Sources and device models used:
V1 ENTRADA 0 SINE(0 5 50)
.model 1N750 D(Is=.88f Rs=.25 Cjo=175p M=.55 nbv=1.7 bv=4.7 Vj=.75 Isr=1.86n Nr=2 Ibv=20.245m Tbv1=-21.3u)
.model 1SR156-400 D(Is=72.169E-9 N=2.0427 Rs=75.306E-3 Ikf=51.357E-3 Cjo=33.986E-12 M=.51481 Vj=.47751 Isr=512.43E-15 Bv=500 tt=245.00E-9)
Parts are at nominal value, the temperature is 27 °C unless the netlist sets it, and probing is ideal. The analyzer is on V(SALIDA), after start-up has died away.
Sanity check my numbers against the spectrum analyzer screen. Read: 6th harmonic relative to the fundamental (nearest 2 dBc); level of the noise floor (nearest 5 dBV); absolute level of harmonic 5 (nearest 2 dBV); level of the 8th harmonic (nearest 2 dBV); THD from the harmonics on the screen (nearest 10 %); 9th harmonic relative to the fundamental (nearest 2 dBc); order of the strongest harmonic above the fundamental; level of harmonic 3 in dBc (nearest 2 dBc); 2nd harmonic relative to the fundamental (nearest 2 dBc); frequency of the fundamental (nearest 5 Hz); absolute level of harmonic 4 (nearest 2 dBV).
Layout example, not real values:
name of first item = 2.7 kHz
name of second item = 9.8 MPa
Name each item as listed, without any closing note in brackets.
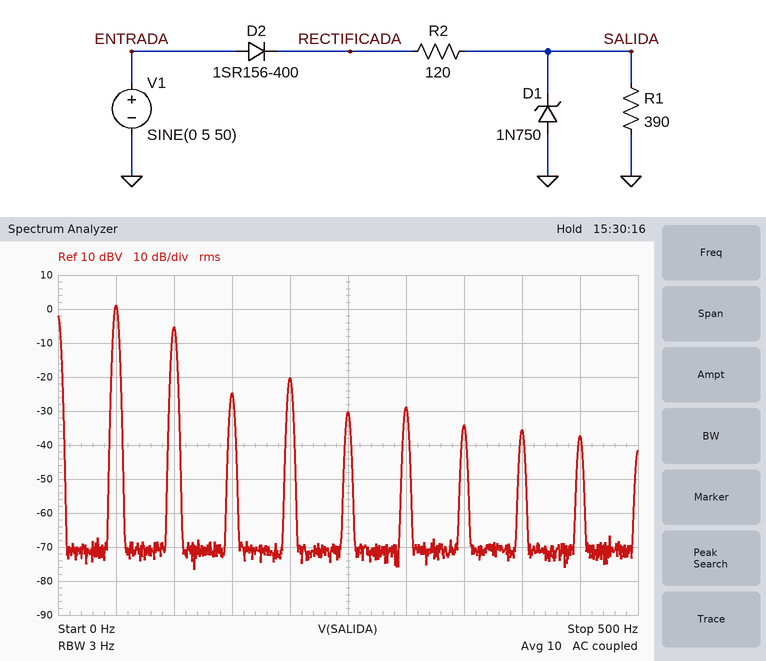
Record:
6th harmonic relative to the fundamental = -30 dBc
level of the noise floor = -70 dBV
absolute level of harmonic 5 = -30 dBV
level of the 8th harmonic = -36 dBV
THD from the harmonics on the screen = 50 %
9th harmonic relative to the fundamental = -38 dBc
order of the strongest harmonic above the fundamental = 2
level of harmonic 3 in dBc = -26 dBc
2nd harmonic relative to the fundamental = -6 dBc
frequency of the fundamental = 50 Hz
absolute level of harmonic 4 = -20 dBV
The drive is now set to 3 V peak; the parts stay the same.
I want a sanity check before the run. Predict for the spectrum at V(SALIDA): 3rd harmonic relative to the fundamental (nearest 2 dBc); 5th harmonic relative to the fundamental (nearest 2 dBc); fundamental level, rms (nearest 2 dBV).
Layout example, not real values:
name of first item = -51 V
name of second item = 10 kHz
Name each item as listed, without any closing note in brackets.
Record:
3rd harmonic relative to the fundamental = -22 dBc
5th harmonic relative to the fundamental = -28 dBc
fundamental level, rms = -4 dBV
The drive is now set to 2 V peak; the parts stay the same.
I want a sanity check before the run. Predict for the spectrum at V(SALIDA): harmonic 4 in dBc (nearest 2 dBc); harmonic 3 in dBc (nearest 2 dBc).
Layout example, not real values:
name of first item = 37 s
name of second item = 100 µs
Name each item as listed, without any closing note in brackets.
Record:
harmonic 4 in dBc = -24 dBc
harmonic 3 in dBc = -18 dBc
